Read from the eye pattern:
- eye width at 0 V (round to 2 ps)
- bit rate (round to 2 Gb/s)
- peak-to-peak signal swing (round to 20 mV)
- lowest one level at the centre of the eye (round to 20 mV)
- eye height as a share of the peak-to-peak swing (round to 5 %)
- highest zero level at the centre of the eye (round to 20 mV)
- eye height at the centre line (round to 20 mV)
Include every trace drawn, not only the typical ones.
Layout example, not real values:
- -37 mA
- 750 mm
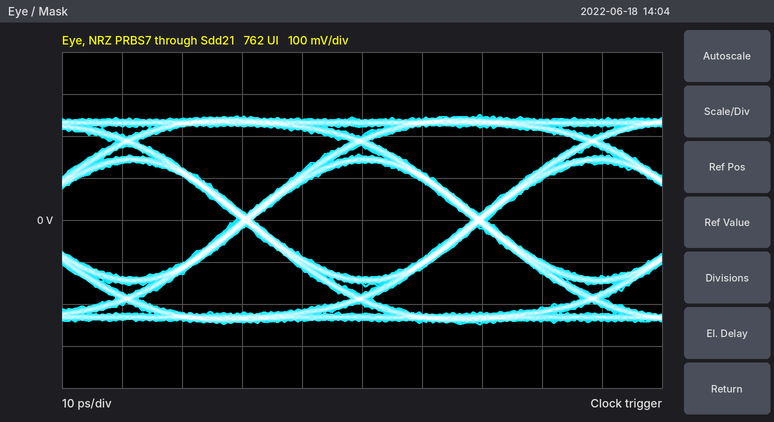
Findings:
- 36 ps
- 26 Gb/s
- 500 mV
- 140 mV
- 55 %
- -140 mV
- 280 mV
